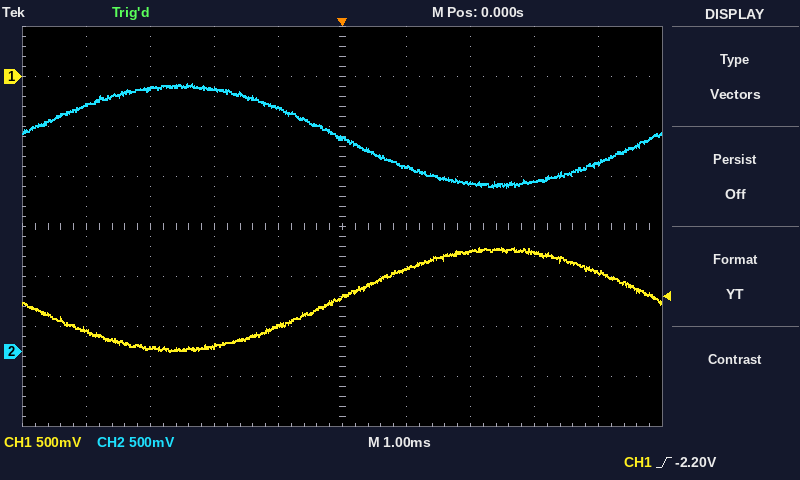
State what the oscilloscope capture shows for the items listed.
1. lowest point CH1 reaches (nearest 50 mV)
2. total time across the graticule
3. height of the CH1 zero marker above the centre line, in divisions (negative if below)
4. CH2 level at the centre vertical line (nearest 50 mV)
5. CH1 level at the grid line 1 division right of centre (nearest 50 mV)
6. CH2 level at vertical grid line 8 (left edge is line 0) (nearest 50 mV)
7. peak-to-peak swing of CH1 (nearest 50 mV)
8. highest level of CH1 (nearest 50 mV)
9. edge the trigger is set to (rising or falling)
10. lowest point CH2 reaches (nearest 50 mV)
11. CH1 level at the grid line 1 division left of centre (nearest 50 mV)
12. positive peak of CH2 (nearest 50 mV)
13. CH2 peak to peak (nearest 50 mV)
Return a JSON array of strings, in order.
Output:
["-2.75 V", "10 ms", "+3.0 div", "2.15 V", "-1.90 V", "1.70 V", "1.05 V", "-1.70 V", "rising", "1.65 V", "-2.50 V", "2.70 V", "1.05 V"]
